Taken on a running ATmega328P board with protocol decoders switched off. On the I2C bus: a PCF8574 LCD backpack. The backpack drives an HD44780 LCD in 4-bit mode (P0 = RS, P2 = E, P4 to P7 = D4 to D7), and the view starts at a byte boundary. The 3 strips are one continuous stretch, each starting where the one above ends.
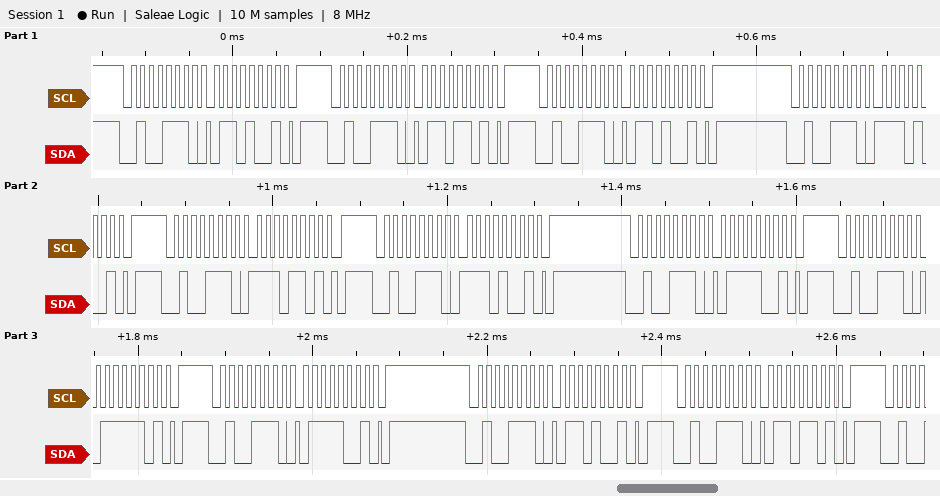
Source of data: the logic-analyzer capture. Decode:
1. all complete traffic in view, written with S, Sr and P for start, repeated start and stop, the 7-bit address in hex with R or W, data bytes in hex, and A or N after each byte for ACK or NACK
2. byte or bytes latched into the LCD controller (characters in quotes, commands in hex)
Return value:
S 27W A 69 A P S 27W A 6D A P S 27W A 69 A P S 27W A E9 A P S 27W A ED A P S 27W A E9 A P S 27W A 79 A P S 27W A 7D A P S 27W A 79 A P S 27W A 69 A P S 27W A 6D A P
'n'
